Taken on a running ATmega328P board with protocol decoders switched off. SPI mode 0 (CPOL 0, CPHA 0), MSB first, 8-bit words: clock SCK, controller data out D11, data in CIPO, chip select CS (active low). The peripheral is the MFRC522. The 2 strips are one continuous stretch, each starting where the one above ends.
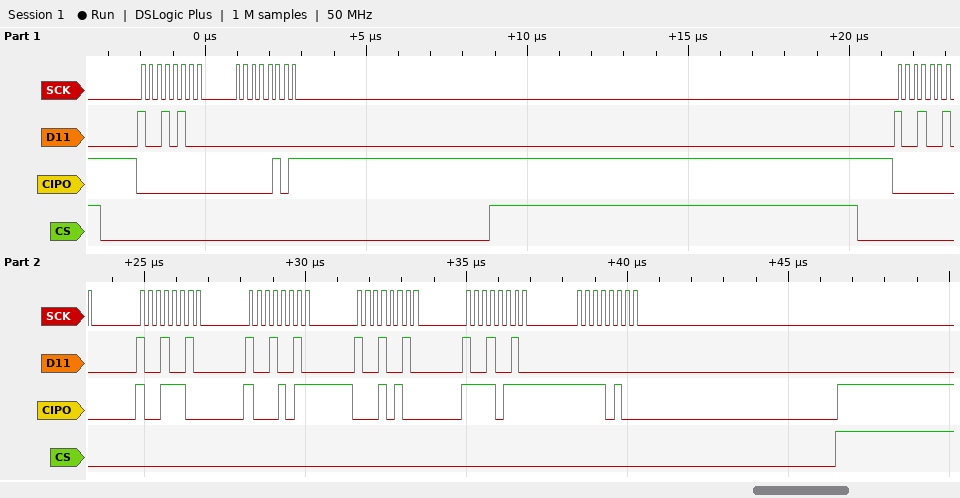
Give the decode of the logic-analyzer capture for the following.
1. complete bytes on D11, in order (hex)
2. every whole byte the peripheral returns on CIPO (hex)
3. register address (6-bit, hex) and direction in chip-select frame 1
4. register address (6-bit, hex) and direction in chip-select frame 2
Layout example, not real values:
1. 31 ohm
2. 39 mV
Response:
1. 0x94 0x00 0x92 0x92 0x92 0x92 0x92 0x00
2. 0x00 0x05 0x00 0x9C 0x8B 0x14 0xF7 0xF4
3. 0x0A read
4. 0x09 read
